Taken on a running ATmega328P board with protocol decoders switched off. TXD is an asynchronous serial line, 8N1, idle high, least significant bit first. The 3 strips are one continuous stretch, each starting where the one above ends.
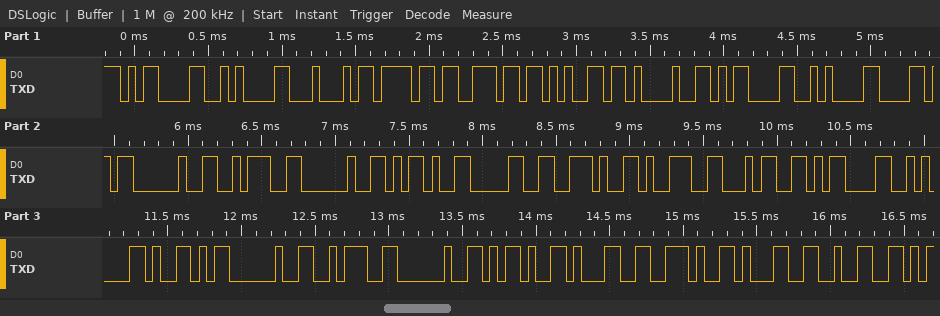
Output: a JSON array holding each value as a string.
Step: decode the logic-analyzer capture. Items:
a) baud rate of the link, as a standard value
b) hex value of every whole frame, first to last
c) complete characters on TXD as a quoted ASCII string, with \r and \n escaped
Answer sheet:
["19200 baud", "0D 0A 44 6F 6E 65 21 0D 0A 58 20 3A 20 2D 30 2E 39 34 0D 0A 59 20 3A 20 2D 31 2E 31 32", "\"\\r\\nDone!\\r\\nX : -0.94\\r\\nY : -1.12\""]
